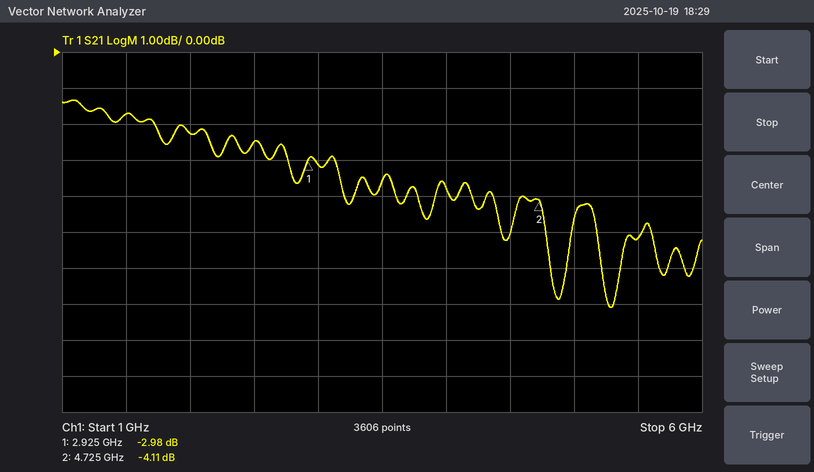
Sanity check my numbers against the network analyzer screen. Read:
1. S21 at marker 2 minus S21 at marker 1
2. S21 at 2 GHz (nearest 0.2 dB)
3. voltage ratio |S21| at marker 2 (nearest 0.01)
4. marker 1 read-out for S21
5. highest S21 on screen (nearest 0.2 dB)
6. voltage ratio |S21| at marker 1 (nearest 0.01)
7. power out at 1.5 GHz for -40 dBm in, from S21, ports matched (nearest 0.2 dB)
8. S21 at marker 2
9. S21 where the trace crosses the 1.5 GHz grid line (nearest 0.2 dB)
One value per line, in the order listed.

-1.13 dB
-2.2 dB
0.62
-2.98 dB
-1.4 dB
0.71
-41.8 dBm
-4.11 dB
-1.8 dB
